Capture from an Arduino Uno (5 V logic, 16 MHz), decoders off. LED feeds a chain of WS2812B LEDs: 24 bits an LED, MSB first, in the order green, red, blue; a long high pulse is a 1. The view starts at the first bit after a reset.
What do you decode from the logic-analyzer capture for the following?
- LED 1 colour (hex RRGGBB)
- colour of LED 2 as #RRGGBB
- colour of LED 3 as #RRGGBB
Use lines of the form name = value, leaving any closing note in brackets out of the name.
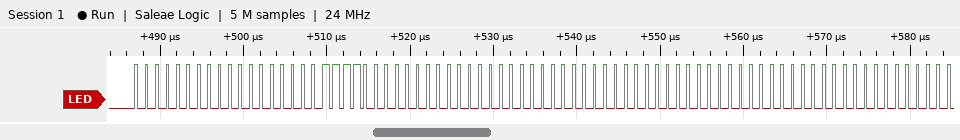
LED 1 colour = #00003C
colour of LED 2 as #RRGGBB = #000000
colour of LED 3 as #RRGGBB = #000000
